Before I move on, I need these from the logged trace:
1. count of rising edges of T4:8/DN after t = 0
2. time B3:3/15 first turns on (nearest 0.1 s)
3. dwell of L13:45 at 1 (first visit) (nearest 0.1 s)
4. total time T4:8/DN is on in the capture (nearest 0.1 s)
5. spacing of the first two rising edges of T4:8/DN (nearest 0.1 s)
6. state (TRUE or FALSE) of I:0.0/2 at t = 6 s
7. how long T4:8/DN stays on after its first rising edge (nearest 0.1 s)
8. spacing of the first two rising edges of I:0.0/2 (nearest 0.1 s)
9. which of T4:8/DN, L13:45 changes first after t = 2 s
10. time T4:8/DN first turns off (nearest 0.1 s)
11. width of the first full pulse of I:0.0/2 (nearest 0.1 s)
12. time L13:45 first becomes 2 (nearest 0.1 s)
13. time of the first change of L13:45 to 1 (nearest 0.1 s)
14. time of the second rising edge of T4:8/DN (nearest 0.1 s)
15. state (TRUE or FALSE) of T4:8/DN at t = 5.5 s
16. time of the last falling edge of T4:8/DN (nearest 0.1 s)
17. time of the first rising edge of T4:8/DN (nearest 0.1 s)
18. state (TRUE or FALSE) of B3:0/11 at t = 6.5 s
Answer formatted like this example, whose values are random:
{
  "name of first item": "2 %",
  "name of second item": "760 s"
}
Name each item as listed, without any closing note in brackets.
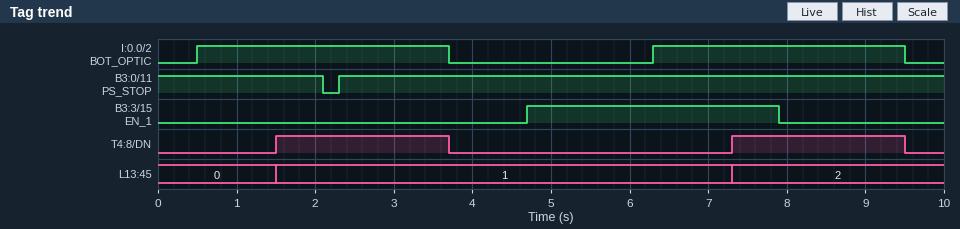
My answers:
{
  "count of rising edges of T4:8/DN after t = 0": "2",
  "time B3:3/15 first turns on": "4.7 s",
  "dwell of L13:45 at 1 (first visit)": "5.8 s",
  "total time T4:8/DN is on in the capture": "4.4 s",
  "spacing of the first two rising edges of T4:8/DN": "5.8 s",
  "state (TRUE or FALSE) of I:0.0/2 at t = 6 s": "FALSE",
  "how long T4:8/DN stays on after its first rising edge": "2.2 s",
  "spacing of the first two rising edges of I:0.0/2": "5.8 s",
  "which of T4:8/DN, L13:45 changes first after t = 2 s": "T4:8/DN",
  "time T4:8/DN first turns off": "3.7 s",
  "width of the first full pulse of I:0.0/2": "3.2 s",
  "time L13:45 first becomes 2": "7.3 s",
  "time of the first change of L13:45 to 1": "1.5 s",
  "time of the second rising edge of T4:8/DN": "7.3 s",
  "state (TRUE or FALSE) of T4:8/DN at t = 5.5 s": "FALSE",
  "time of the last falling edge of T4:8/DN": "9.5 s",
  "time of the first rising edge of T4:8/DN": "1.5 s",
  "state (TRUE or FALSE) of B3:0/11 at t = 6.5 s": "TRUE"
}
